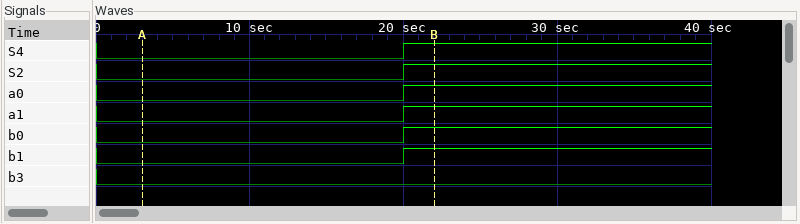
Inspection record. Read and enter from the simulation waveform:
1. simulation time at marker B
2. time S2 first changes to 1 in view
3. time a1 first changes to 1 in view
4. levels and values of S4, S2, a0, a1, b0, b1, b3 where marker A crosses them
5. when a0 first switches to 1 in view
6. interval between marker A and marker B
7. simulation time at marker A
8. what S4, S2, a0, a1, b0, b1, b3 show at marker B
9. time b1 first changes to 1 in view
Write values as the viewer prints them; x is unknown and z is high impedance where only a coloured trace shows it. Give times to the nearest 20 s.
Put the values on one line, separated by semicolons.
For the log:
20 s; 20 s; 20 s; S4=0, S2=0, a0=0, a1=0, b0=0, b1=0, b3=0; 20 s; 20 s; 0 s; S4=1, S2=1, a0=1, a1=1, b0=1, b1=1, b3=0; 20 s
